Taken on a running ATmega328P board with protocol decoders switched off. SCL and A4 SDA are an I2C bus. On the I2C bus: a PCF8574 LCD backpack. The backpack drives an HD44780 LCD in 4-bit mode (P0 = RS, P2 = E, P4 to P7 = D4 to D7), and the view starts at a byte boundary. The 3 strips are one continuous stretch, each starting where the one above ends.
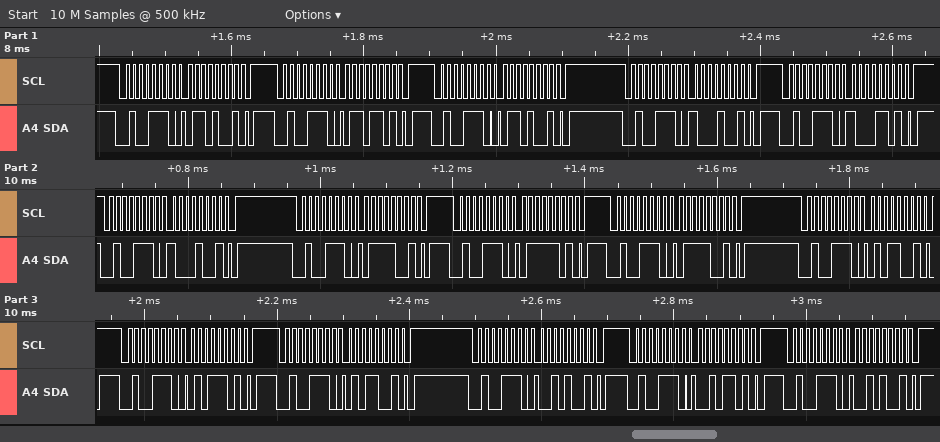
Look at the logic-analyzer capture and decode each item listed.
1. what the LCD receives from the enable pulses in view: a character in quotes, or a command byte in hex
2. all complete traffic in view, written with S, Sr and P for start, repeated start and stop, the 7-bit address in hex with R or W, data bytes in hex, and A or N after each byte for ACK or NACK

'h' 'u'
S 27W A 69 A P S 27W A 6D A P S 27W A 69 A P S 27W A 89 A P S 27W A 8D A P S 27W A 89 A P S 27W A 79 A P S 27W A 7D A P S 27W A 79 A P S 27W A 59 A P S 27W A 5D A P S 27W A 59 A P S 27W A 29 A P S 27W A 2D A P S 27W A 29 A P
